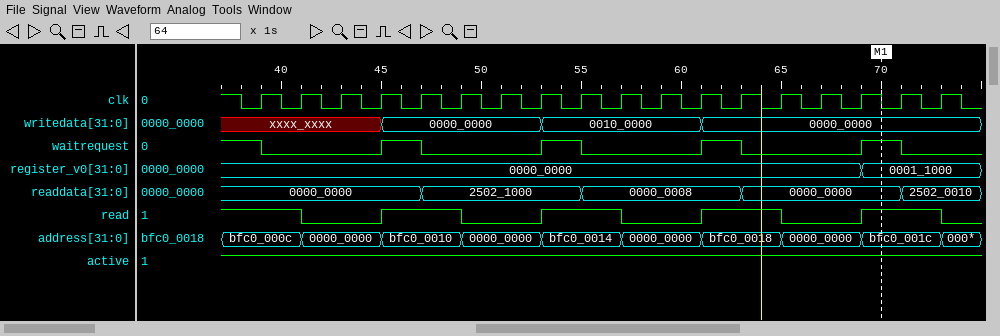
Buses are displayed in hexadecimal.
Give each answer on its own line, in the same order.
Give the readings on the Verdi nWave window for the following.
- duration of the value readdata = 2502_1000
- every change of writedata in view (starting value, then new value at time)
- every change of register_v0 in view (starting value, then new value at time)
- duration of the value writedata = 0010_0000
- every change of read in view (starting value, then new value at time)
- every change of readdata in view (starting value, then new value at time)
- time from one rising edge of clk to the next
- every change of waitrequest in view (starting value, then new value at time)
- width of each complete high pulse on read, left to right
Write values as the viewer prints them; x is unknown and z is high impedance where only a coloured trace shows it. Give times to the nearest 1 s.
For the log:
8 s
xxxx_xxxx, 0000_0000 at 45 s, 0010_0000 at 53 s, 0000_0000 at 61 s
0000_0000, 0001_1000 at 69 s
8 s
1, 0 at 41 s, 1 at 45 s, 0 at 49 s, 1 at 53 s, 0 at 57 s, 1 at 61 s, 0 at 65 s, 1 at 69 s, 0 at 73 s
0000_0000, 2502_1000 at 47 s, 0000_0008 at 55 s, 0000_0000 at 63 s, 2502_0010 at 71 s
2 s
1, 0 at 39 s, 1 at 45 s, 0 at 47 s, 1 at 53 s, 0 at 55 s, 1 at 61 s, 0 at 63 s, 1 at 69 s, 0 at 71 s
4 s, 4 s, 4 s, 4 s
